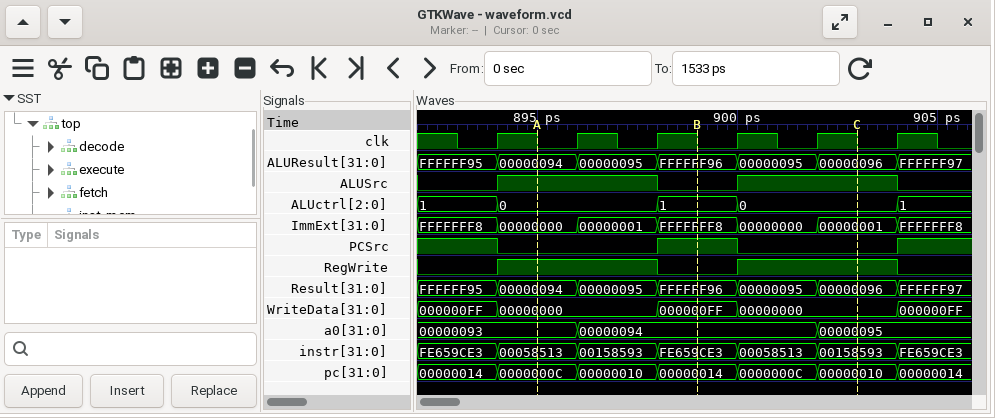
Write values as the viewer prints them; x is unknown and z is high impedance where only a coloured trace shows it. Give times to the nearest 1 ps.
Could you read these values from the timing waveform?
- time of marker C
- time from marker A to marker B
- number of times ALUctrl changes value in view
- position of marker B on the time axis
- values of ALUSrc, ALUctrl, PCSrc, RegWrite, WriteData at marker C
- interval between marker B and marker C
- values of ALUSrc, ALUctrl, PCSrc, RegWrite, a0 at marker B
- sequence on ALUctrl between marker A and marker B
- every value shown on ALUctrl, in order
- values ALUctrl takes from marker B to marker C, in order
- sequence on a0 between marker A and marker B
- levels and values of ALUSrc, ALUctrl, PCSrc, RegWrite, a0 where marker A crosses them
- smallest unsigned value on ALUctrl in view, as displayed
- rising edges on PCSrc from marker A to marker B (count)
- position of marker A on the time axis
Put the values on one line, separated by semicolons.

903 ps; 4 ps; 4; 899 ps; ALUSrc=1, ALUctrl=0, PCSrc=0, RegWrite=1, WriteData=00000000; 4 ps; ALUSrc=0, ALUctrl=1, PCSrc=1, RegWrite=0, a0=00000094; 0, 1; 1, 0, 1, 0, 1; 1, 0; 00000093, 00000094; ALUSrc=1, ALUctrl=0, PCSrc=0, RegWrite=1, a0=00000093; 0; 1; 895 ps
